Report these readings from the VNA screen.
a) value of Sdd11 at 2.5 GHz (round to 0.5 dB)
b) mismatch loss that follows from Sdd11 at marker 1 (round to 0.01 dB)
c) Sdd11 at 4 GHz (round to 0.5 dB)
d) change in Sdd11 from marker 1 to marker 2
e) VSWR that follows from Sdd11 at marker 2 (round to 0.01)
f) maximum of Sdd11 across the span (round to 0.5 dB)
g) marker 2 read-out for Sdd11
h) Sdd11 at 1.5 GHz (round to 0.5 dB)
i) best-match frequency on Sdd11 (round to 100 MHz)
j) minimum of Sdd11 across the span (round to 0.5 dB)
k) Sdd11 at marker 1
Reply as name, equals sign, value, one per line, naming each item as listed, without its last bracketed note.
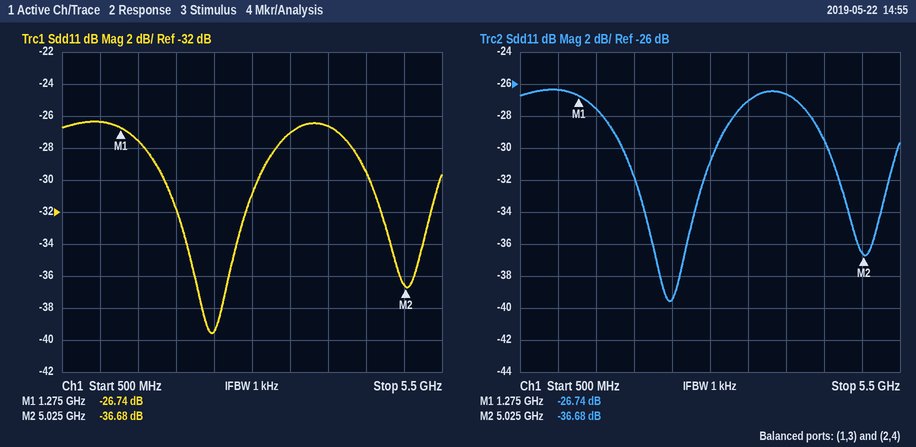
value of Sdd11 at 2.5 GHz = -39.5 dB
mismatch loss that follows from Sdd11 at marker 1 = 0.01 dB
Sdd11 at 4 GHz = -26.5 dB
change in Sdd11 from marker 1 to marker 2 = -9.94 dB
VSWR that follows from Sdd11 at marker 2 = 1.03
maximum of Sdd11 across the span = -26.5 dB
marker 2 read-out for Sdd11 = -36.68 dB
Sdd11 at 1.5 GHz = -27.5 dB
best-match frequency on Sdd11 = 2.5 GHz
minimum of Sdd11 across the span = -39.5 dB
Sdd11 at marker 1 = -26.74 dB
